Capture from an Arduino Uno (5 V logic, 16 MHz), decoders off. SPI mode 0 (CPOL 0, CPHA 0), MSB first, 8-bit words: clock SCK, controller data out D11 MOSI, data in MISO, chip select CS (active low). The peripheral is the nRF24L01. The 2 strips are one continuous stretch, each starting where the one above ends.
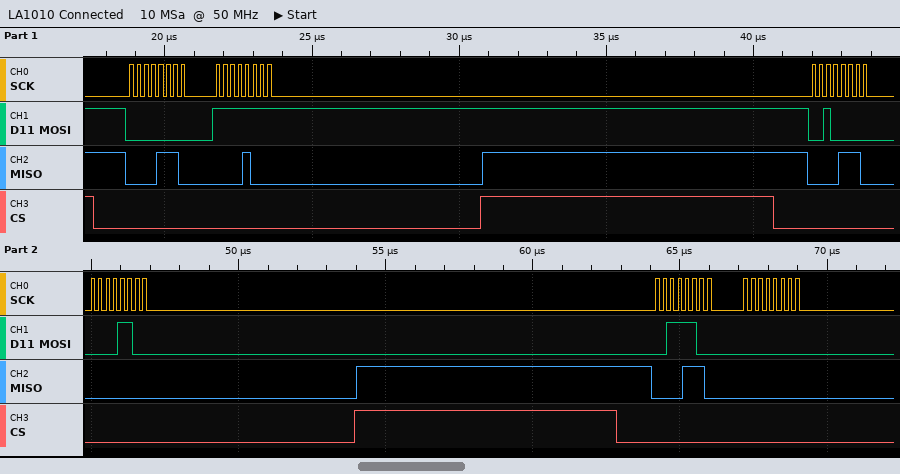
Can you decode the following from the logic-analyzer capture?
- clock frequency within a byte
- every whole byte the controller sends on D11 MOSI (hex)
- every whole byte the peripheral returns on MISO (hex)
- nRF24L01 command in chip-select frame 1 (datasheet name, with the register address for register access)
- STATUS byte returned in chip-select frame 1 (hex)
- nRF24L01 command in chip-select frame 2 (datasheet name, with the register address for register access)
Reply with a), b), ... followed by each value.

a) 4 MHz
b) 00 FF 20 0C 3C 00
c) 0E 08 0E 00 0E 00
d) R_REGISTER 0x00
e) 0x0E
f) W_REGISTER 0x00
